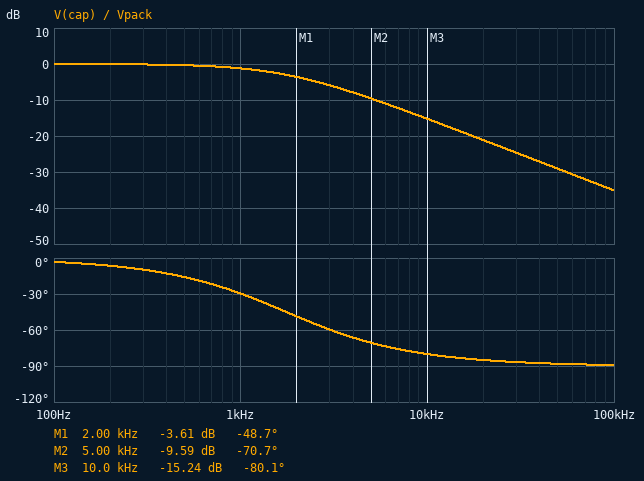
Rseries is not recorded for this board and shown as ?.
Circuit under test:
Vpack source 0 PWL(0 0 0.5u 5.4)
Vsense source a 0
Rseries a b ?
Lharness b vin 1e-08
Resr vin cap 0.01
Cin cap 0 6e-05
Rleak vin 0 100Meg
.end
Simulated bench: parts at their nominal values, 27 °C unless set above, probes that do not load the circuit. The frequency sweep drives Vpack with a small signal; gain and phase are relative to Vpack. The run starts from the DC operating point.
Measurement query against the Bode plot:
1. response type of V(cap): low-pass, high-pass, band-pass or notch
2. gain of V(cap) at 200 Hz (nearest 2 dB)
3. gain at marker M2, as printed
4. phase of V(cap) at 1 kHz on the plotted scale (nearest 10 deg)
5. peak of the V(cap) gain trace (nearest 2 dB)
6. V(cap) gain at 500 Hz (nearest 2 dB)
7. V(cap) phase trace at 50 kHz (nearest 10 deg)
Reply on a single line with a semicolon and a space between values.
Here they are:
low-pass; 0 dB; -9.59 dB; -30 deg; 0 dB; 0 dB; -90 deg
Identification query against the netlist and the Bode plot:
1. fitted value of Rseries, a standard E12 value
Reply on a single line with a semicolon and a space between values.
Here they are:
1.5 Ω
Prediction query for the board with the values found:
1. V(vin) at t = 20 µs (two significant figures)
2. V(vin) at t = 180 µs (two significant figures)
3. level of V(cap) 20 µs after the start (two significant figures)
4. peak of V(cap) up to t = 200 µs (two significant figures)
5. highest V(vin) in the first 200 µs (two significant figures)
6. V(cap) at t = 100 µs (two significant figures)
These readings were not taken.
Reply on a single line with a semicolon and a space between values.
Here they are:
1.1 V; 4.7 V; 1.1 V; 4.8 V; 4.8 V; 3.6 V
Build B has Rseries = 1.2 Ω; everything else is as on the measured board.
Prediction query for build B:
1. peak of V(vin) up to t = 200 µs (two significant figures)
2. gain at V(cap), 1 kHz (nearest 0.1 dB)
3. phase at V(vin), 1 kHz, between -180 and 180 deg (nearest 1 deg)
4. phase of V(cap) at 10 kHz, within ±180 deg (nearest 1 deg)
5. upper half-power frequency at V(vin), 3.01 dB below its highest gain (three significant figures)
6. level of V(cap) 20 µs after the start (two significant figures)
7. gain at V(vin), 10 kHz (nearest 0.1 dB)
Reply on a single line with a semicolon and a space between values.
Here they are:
5.1 V; -0.8 dB; -24 deg; -78 deg; 2.19 kHz; 1.3 V; -13.4 dB
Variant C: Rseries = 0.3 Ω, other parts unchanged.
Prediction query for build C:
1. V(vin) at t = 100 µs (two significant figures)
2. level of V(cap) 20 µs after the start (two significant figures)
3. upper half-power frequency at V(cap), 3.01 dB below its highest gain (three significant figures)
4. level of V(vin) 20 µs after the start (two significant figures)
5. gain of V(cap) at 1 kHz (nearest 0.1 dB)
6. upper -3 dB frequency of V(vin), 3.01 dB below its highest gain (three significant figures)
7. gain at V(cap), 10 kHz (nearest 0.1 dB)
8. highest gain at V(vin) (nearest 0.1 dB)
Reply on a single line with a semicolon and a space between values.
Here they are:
5.4 V; 3.5 V; 8.57 kHz; 3.6 V; -0.1 dB; 8.58 kHz; -3.7 dB; 0 dB
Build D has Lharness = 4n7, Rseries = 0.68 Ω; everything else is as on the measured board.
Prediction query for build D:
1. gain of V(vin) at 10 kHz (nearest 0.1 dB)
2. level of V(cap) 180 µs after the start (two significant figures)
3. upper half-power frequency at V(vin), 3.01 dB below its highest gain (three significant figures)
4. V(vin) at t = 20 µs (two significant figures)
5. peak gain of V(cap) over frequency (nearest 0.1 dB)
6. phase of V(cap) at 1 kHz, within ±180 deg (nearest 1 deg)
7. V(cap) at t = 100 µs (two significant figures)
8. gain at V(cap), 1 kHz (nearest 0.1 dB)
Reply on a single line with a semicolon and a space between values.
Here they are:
-8.9 dB; 5.3 V; 3.85 kHz; 2.1 V; 0 dB; -15 deg; 4.9 V; -0.3 dB
